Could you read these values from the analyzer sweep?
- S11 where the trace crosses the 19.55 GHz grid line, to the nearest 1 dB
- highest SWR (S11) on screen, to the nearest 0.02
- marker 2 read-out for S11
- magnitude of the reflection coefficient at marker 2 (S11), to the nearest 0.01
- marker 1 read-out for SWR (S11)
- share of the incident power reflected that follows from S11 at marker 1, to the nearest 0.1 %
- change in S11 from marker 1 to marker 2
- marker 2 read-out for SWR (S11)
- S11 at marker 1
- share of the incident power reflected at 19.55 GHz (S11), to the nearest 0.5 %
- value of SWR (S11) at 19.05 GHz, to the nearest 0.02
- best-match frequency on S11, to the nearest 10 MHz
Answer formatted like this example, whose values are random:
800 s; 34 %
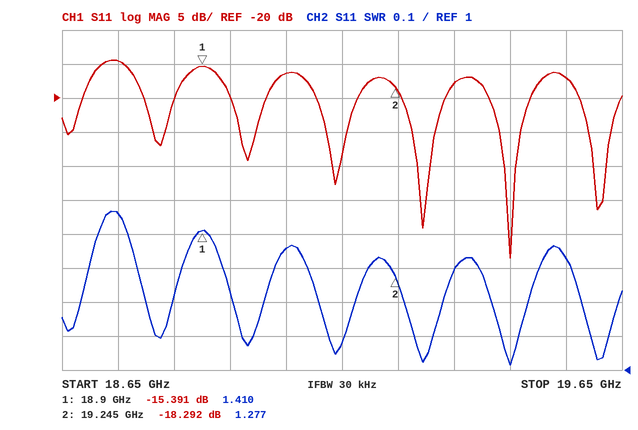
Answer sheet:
-17 dB; 1.46; -18.292 dB; 0.12; 1.410; 2.9 %; -2.901 dB; 1.277; -15.391 dB; 2.0 %; 1.36; 19.45 GHz
